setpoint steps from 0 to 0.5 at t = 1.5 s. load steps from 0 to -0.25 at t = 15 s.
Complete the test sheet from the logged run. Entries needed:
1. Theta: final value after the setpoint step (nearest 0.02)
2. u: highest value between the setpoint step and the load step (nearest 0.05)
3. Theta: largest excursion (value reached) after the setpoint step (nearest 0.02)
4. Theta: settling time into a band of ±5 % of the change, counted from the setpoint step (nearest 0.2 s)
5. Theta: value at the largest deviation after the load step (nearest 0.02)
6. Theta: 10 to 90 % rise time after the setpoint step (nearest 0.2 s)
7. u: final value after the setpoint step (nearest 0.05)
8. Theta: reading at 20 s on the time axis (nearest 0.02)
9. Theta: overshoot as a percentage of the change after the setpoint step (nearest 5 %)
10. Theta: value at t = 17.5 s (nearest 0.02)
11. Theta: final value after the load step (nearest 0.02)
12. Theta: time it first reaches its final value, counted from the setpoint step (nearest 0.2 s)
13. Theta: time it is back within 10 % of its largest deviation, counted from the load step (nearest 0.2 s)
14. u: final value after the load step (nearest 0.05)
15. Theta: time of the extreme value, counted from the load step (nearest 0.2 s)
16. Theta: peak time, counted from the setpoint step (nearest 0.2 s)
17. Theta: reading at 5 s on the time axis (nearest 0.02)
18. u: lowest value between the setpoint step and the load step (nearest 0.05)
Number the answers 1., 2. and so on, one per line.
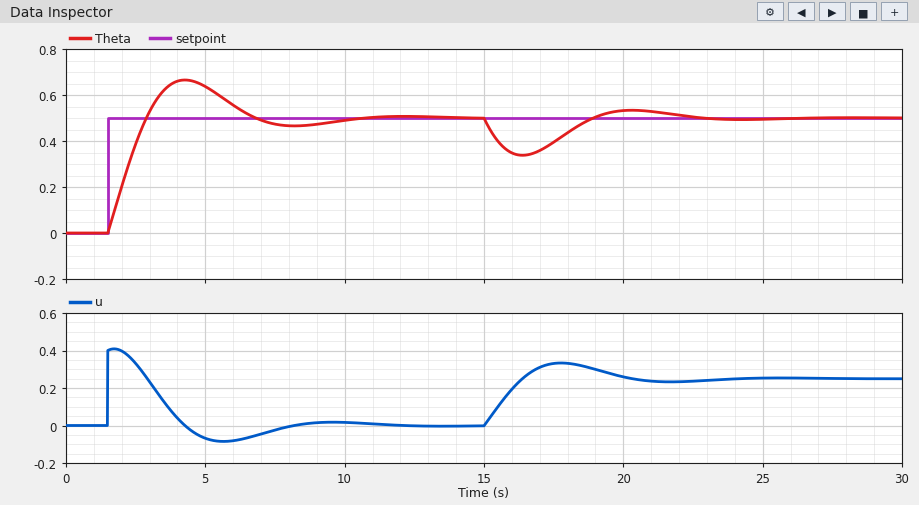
1. 0.50
2. 0.40
3. 0.66
4. 7.6 s
5. 0.34
6. 1.0 s
7. 0.00
8. 0.54
9. 35 %
10. 0.40
11. 0.50
12. 1.4 s
13. 6.8 s
14. 0.25
15. 1.4 s
16. 2.8 s
17. 0.64
18. -0.10
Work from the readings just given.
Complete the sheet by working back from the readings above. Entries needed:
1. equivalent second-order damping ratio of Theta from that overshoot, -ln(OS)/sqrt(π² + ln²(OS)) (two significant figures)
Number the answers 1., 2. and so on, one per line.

1. 0.32
